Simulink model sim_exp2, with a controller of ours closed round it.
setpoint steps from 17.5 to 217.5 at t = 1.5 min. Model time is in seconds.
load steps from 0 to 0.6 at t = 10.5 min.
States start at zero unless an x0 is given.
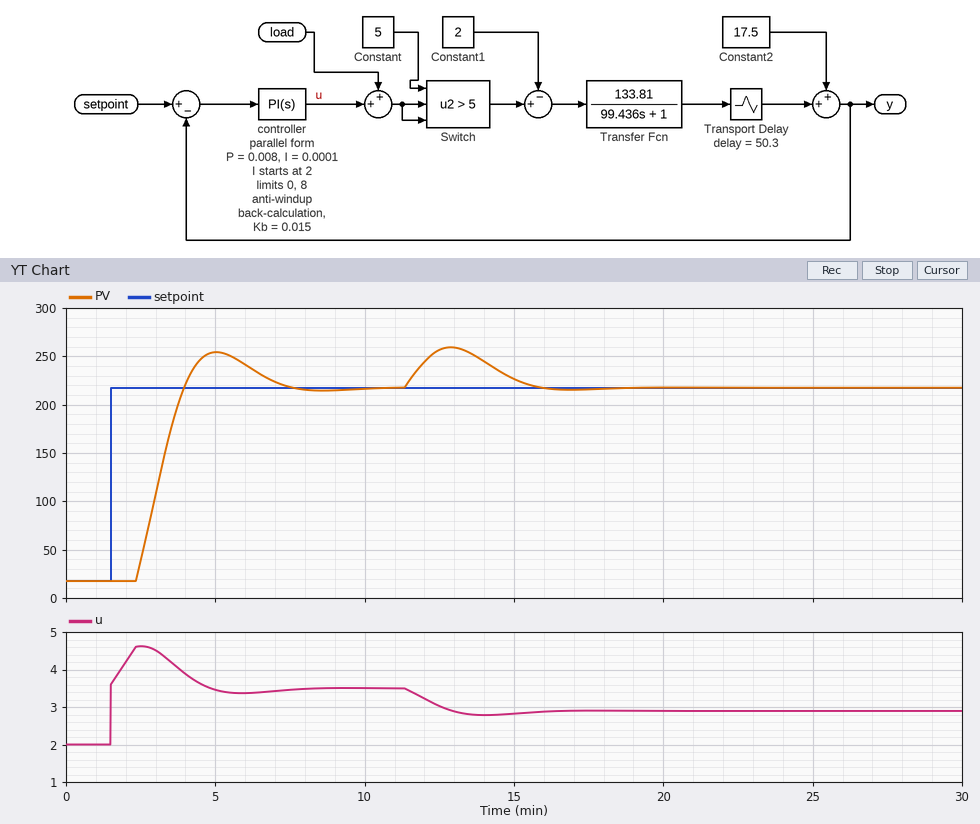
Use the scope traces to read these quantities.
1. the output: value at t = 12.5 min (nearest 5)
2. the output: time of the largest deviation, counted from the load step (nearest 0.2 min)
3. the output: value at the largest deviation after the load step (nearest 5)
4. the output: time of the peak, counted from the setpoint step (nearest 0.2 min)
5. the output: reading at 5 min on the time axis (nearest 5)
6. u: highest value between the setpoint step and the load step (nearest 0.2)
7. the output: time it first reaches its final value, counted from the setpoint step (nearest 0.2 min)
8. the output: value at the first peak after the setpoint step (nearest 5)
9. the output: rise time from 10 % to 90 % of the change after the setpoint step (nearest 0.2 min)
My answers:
255
2.4 min
260
3.6 min
255
4.6
2.4 min
255
1.2 min
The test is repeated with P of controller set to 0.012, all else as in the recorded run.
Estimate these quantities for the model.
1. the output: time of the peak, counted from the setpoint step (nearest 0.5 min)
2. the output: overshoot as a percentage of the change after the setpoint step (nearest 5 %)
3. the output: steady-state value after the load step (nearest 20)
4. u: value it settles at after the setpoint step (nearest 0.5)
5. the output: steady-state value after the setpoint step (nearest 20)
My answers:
3.0 min
20 %
220
3.5
220
